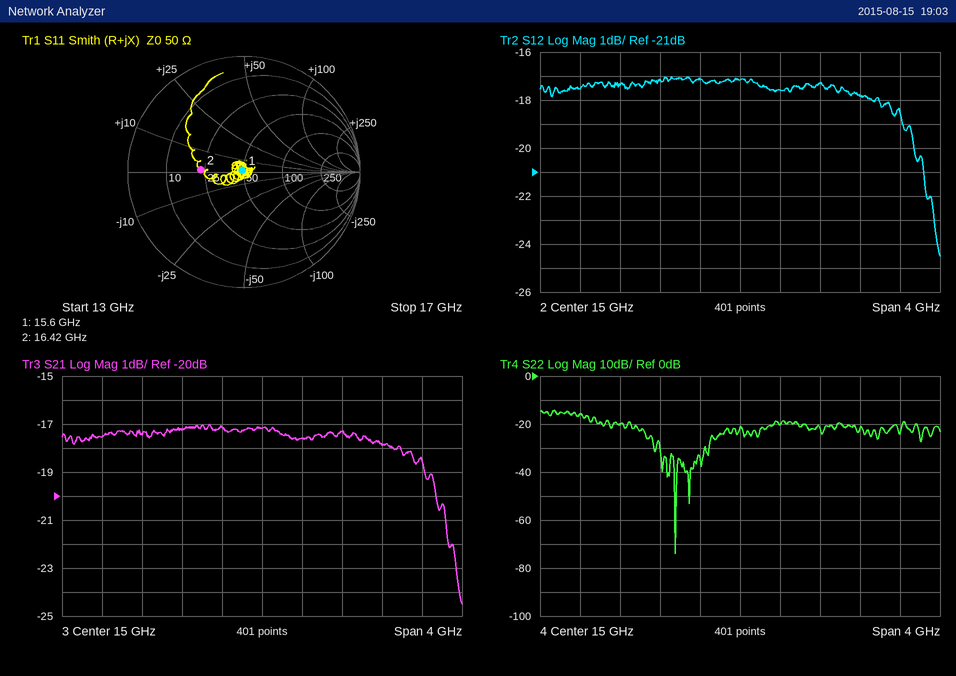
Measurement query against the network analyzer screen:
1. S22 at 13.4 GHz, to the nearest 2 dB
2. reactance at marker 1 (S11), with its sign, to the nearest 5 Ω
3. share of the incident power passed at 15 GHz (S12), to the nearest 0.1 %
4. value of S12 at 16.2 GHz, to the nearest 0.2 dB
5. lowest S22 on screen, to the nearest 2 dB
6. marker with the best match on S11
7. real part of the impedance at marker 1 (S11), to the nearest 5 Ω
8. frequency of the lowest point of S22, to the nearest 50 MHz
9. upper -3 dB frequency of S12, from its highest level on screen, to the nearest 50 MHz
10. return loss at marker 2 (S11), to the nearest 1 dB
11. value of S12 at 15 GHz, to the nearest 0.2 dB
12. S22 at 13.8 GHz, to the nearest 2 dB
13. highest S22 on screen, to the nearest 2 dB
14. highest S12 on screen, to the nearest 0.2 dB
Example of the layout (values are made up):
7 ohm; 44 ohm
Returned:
-16 dB; 0 Ω; 1.9 %; -17.8 dB; -74 dB; marker 1; 50 Ω; 14.35 GHz; 16.75 GHz; 9 dB; -17.2 dB; -20 dB; -14 dB; -17.0 dB
